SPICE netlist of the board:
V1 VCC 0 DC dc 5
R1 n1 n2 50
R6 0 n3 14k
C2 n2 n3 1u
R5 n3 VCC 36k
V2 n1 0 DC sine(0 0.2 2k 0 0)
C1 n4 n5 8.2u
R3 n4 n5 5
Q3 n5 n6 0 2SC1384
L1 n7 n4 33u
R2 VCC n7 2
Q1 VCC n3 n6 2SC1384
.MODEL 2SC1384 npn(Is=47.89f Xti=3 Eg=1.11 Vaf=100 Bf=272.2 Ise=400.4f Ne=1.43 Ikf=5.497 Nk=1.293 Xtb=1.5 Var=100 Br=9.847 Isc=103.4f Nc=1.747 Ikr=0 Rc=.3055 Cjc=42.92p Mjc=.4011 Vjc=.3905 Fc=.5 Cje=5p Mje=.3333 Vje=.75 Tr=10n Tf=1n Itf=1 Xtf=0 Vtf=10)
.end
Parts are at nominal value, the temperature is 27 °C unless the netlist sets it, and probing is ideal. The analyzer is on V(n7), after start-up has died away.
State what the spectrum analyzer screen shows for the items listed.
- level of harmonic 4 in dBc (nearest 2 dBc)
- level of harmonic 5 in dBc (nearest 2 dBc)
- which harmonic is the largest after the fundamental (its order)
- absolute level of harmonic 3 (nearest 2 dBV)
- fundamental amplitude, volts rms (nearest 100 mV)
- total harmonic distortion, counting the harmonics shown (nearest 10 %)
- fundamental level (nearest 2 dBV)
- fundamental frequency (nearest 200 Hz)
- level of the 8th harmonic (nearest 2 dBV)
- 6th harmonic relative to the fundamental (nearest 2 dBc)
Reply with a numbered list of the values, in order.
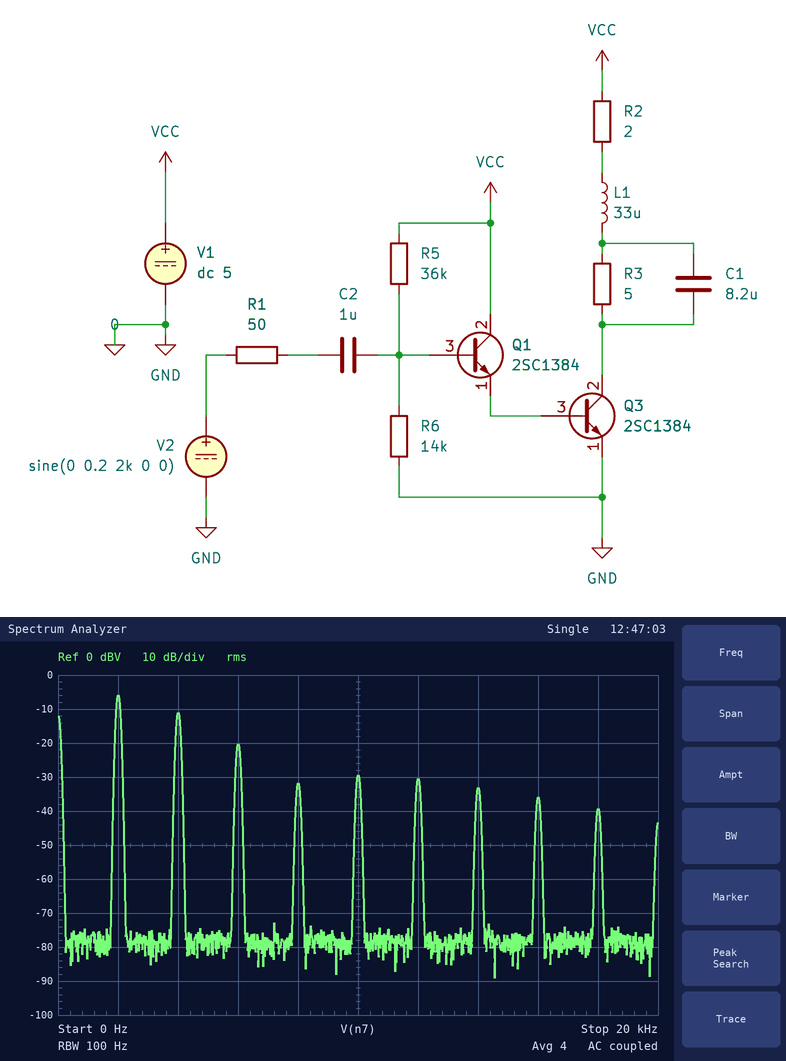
1. -26 dBc
2. -24 dBc
3. 2
4. -20 dBV
5. 500 mV
6. 60 %
7. -6 dBV
8. 2.0 kHz
9. -36 dBV
10. -24 dBc
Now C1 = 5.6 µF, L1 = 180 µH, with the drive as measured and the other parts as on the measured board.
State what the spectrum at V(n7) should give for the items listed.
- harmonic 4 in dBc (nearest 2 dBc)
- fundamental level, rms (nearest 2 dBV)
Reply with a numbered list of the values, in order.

1. -38 dBc
2. -6 dBV
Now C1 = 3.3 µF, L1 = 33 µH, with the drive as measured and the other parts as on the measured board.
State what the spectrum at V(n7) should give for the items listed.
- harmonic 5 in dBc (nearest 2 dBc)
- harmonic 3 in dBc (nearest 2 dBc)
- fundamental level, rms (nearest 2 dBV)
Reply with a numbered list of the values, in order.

1. -20 dBc
2. -16 dBc
3. -6 dBV
